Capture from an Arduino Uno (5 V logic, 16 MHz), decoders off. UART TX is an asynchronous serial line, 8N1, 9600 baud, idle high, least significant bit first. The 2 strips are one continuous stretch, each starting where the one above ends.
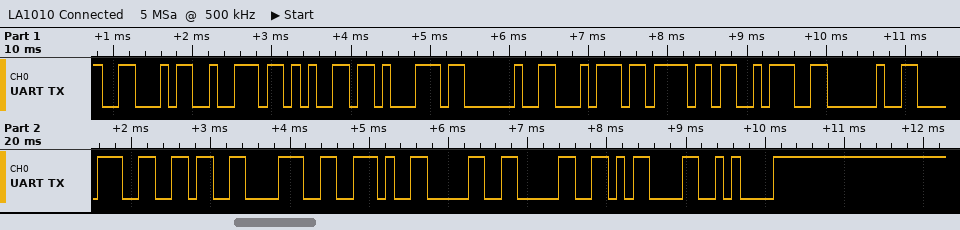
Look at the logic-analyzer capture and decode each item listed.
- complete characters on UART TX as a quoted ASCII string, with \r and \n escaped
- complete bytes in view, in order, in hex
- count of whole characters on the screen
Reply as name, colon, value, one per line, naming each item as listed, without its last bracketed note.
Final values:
complete characters on UART TX as a quoted ASCII string, with \r and \n escaped: "Freq to: 868.00\r\n"
complete bytes in view, in order, in hex: 0x46 0x72 0x65 0x71 0x20 0x74 0x6F 0x3A 0x20 0x38 0x36 0x38 0x2E 0x30 0x30 0x0D 0x0A
count of whole characters on the screen: 17
